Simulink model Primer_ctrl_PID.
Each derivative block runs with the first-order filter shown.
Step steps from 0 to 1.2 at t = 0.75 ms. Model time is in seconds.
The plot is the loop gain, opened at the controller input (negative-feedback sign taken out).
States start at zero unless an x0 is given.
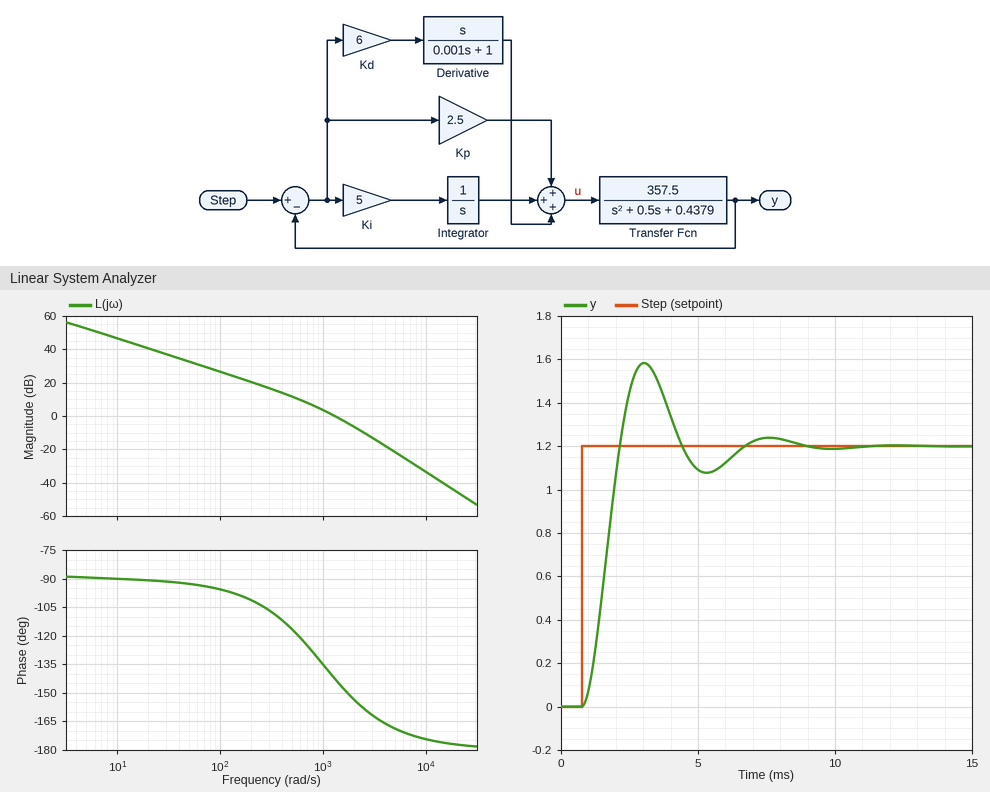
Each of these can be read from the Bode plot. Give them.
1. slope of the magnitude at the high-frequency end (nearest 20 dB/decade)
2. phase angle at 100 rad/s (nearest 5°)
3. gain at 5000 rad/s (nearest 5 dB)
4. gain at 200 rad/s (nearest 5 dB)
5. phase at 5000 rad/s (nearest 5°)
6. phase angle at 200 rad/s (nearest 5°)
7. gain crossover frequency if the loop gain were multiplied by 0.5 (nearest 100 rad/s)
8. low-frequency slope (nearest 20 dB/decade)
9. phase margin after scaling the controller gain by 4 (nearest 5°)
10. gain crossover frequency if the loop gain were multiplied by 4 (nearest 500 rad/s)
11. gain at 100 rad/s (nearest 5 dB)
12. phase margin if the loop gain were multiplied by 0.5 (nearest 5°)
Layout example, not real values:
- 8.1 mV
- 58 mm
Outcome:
- -40 dB/decade
- -95°
- -20 dB
- 20 dB
- -170°
- -100°
- 800 rad/s
- -20 dB/decade
- 20°
- 3000 rad/s
- 25 dB
- 50°
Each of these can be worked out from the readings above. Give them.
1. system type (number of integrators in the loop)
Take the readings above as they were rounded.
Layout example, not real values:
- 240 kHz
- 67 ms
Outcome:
- 1
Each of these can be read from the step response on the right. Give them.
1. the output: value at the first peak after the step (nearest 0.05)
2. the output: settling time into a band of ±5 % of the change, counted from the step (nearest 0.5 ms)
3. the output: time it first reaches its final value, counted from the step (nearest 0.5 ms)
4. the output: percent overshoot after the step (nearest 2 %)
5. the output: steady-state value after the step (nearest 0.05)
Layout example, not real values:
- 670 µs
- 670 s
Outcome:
- 1.60
- 5.5 ms
- 1.5 ms
- 32 %
- 1.20
